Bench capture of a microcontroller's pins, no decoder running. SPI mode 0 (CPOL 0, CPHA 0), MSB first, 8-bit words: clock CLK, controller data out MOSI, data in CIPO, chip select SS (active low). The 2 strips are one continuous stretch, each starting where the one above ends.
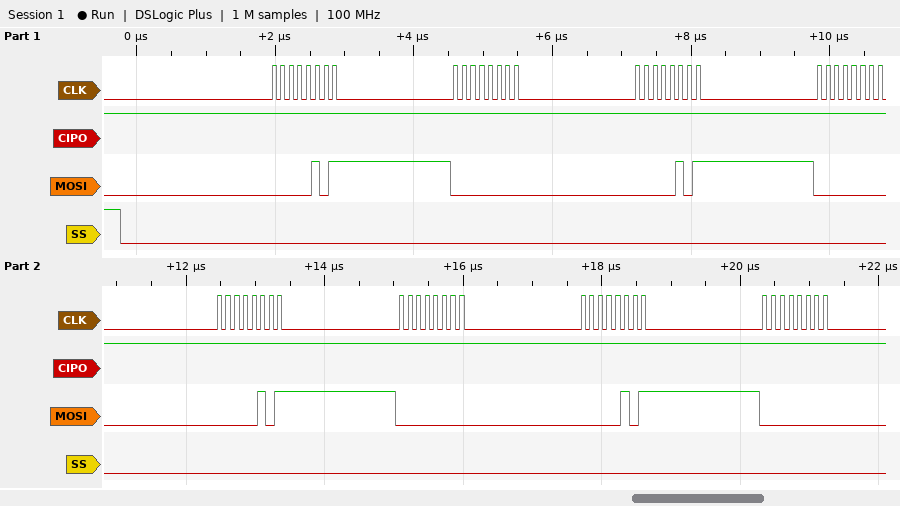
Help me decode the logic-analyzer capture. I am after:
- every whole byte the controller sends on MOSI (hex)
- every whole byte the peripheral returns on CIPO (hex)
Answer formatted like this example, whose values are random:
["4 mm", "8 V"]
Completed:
["05 00 05 00 05 00 05 00", "FF FF FF FF FF FF FF FF"]
